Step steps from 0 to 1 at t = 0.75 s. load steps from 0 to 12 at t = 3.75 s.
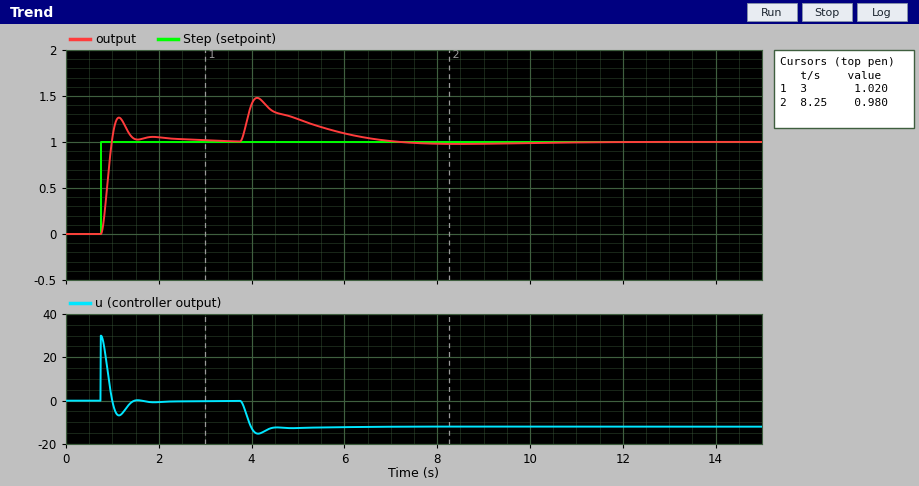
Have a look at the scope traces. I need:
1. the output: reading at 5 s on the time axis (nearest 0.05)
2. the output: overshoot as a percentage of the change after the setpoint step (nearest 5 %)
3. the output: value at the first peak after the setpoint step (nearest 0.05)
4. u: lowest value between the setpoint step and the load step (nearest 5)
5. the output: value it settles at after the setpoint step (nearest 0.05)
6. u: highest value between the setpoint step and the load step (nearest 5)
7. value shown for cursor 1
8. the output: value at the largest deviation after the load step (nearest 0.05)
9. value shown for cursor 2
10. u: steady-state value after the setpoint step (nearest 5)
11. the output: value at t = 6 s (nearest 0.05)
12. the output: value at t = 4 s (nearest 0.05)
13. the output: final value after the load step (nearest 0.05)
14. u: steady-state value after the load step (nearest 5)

1.25
25 %
1.25
-5
1.00
30
1.020
1.50
0.980
0
1.10
1.40
1.00
-10
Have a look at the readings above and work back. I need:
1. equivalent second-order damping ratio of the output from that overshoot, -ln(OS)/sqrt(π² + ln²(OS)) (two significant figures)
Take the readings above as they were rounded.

0.40
